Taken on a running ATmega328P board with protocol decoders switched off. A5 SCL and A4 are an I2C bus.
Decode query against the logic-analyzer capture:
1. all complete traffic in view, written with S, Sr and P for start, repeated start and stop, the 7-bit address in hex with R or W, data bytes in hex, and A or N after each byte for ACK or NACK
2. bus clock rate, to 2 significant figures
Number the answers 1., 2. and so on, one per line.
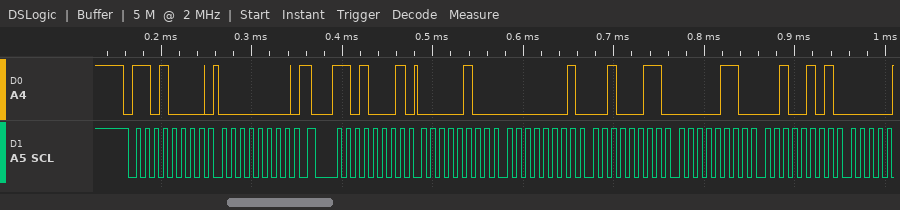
1. S 68W A 00 A Sr 68R A 04 A 01 A 23 A 06 A 25 A
2. 100 kHz
